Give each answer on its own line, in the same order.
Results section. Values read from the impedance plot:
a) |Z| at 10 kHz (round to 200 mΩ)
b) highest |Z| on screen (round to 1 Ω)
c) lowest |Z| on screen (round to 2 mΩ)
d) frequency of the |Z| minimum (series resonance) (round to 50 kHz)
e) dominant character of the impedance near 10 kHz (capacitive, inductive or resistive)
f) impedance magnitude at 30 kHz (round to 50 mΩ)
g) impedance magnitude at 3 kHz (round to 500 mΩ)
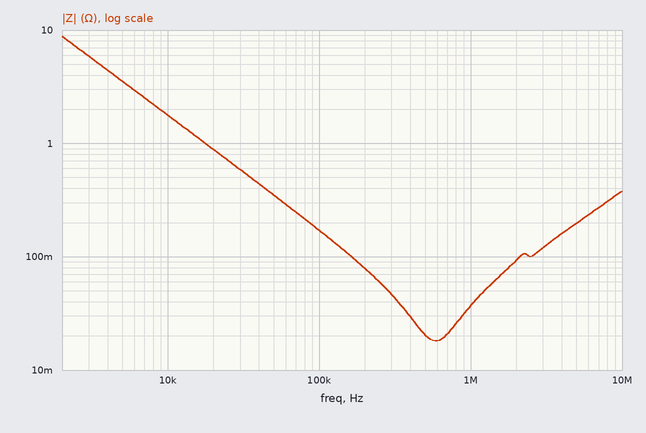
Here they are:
1.8 Ω
9 Ω
18 mΩ
600 kHz
capacitive
600 mΩ
6.0 Ω
